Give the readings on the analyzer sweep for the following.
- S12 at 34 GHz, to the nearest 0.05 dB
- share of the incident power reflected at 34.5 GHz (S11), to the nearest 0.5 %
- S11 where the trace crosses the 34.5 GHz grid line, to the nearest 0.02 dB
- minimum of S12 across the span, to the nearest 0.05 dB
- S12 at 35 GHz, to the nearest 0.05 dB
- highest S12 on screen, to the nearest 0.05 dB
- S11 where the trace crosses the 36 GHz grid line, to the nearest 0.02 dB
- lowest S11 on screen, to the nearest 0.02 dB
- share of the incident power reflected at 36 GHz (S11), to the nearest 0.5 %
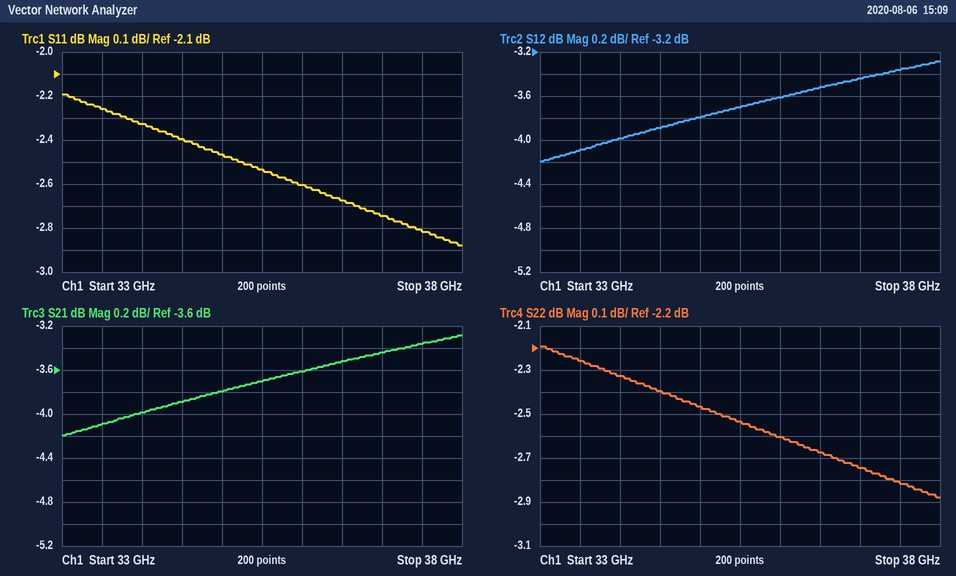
-4.00 dB
57.5 %
-2.40 dB
-4.20 dB
-3.80 dB
-3.30 dB
-2.60 dB
-2.88 dB
55.0 %
